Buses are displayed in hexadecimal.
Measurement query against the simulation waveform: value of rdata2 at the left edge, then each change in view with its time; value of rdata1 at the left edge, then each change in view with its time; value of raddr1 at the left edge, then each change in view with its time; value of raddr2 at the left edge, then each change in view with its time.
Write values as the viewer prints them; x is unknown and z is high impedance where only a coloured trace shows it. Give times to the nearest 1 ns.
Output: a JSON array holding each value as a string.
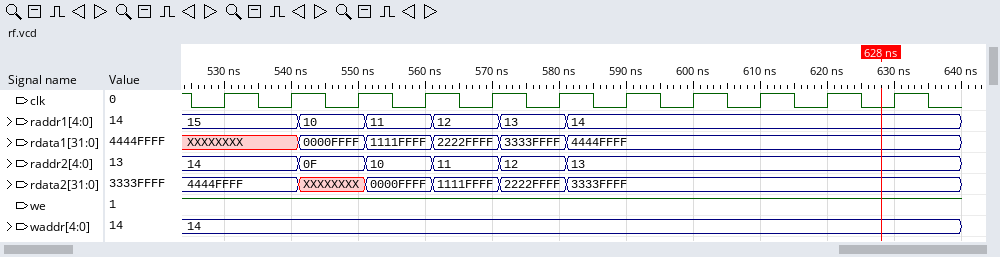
["4444FFFF, XXXXXXXX at 541 ns, 0000FFFF at 551 ns, 1111FFFF at 561 ns, 2222FFFF at 571 ns, 3333FFFF at 581 ns", "XXXXXXXX, 0000FFFF at 541 ns, 1111FFFF at 551 ns, 2222FFFF at 561 ns, 3333FFFF at 571 ns, 4444FFFF at 581 ns", "15, 10 at 541 ns, 11 at 551 ns, 12 at 561 ns, 13 at 571 ns, 14 at 581 ns", "14, 0F at 541 ns, 10 at 551 ns, 11 at 561 ns, 12 at 571 ns, 13 at 581 ns"]
